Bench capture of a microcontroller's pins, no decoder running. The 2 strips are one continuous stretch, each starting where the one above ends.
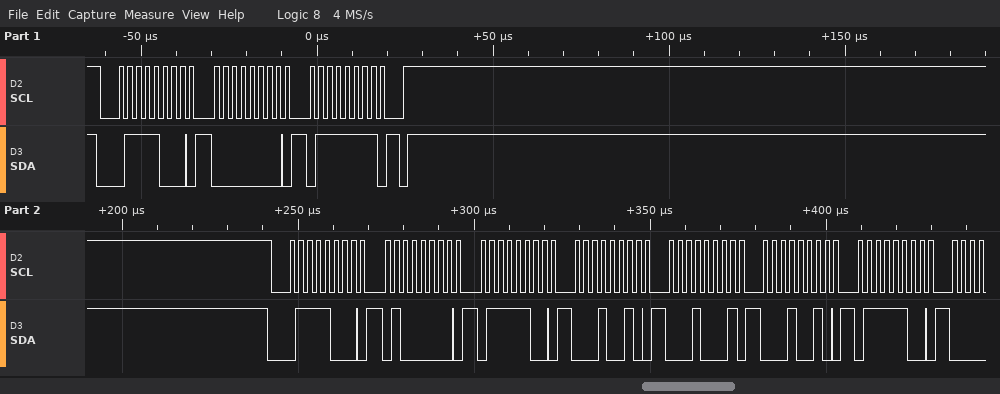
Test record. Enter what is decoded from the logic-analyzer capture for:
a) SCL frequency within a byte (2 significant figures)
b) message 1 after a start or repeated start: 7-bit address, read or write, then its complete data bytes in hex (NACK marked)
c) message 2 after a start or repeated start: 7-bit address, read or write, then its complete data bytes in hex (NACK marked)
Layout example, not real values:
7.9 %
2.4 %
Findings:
400 kHz
0x3C write: 00 7F
0x3C write: 40 7C 12 11 12 7C
